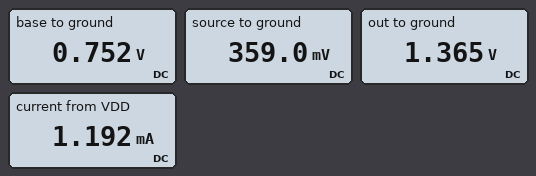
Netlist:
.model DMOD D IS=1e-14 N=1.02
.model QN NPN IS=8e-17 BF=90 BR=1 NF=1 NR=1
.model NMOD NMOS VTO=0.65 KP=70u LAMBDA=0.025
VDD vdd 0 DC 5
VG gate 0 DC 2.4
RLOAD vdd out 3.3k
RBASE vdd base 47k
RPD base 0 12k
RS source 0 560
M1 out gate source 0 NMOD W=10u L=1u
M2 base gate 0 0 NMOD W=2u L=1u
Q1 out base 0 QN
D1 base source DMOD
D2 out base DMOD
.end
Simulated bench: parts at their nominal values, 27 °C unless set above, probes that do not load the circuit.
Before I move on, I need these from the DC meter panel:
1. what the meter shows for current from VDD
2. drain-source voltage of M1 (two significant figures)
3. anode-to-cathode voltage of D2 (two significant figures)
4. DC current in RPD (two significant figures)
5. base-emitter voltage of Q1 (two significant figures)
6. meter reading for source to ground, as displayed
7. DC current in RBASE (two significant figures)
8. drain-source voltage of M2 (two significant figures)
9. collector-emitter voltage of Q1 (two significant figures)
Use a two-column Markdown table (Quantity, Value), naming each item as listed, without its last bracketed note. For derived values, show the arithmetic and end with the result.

| Quantity | Value |
|---|---|
| what the meter shows for current from VDD | 1.192 mA |
| drain-source voltage of M1 | 1.365 V - 359 mV = 1.0 V |
| anode-to-cathode voltage of D2 | 1.365 V - 752 mV = 610 mV |
| DC current in RPD | (752 mV) / 12 kΩ = 63 µA |
| base-emitter voltage of Q1 | 752 mV = 750 mV |
| meter reading for source to ground, as displayed | 359.0 mV |
| DC current in RBASE | (5 V - 752 mV) / 47 kΩ = 90 µA |
| drain-source voltage of M2 | 752 mV = 750 mV |
| collector-emitter voltage of Q1 | 1.365 V = 1.4 V |
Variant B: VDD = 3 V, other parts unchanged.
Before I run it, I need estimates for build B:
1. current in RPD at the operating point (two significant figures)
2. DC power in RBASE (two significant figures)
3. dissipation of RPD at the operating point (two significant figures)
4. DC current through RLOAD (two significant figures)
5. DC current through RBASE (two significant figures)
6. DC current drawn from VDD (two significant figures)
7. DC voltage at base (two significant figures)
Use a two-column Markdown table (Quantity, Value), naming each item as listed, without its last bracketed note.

| Quantity | Value |
|---|---|
| current in RPD at the operating point | 33 µA |
| DC power in RBASE | 140 µW |
| dissipation of RPD at the operating point | 13 µW |
| DC current through RLOAD | 610 µA |
| DC current through RBASE | 55 µA |
| DC current drawn from VDD | 660 µA |
| DC voltage at base | 400 mV |
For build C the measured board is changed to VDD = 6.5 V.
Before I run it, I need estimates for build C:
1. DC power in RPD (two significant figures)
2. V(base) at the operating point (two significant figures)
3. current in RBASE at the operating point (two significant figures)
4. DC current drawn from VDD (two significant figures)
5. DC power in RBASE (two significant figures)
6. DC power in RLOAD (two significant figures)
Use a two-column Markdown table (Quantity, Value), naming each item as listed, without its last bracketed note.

| Quantity | Value |
|---|---|
| DC power in RPD | 50 µW |
| V(base) at the operating point | 770 mV |
| current in RBASE at the operating point | 120 µA |
| DC current drawn from VDD | 1.7 mA |
| DC power in RBASE | 700 µW |
| DC power in RLOAD | 7.9 mW |
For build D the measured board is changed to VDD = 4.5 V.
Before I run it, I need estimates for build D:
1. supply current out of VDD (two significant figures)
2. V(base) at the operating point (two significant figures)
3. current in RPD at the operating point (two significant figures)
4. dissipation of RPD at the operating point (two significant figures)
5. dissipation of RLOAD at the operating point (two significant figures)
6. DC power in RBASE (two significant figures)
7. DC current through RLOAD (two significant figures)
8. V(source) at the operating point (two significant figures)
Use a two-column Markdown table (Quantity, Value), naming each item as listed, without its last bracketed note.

| Quantity | Value |
|---|---|
| supply current out of VDD | 1.0 mA |
| V(base) at the operating point | 740 mV |
| current in RPD at the operating point | 61 µA |
| dissipation of RPD at the operating point | 45 µW |
| dissipation of RLOAD at the operating point | 3.0 mW |
| DC power in RBASE | 300 µW |
| DC current through RLOAD | 950 µA |
| V(source) at the operating point | 360 mV |
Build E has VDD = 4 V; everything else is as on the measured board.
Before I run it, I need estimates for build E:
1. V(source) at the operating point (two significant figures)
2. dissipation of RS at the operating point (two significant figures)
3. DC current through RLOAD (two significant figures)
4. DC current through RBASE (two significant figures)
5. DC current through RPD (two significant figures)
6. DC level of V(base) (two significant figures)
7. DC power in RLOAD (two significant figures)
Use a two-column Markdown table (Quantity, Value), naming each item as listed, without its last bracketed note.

| Quantity | Value |
|---|---|
| V(source) at the operating point | 350 mV |
| dissipation of RS at the operating point | 220 µW |
| DC current through RLOAD | 810 µA |
| DC current through RBASE | 70 µA |
| DC current through RPD | 59 µA |
| DC level of V(base) | 700 mV |
| DC power in RLOAD | 2.2 mW |
